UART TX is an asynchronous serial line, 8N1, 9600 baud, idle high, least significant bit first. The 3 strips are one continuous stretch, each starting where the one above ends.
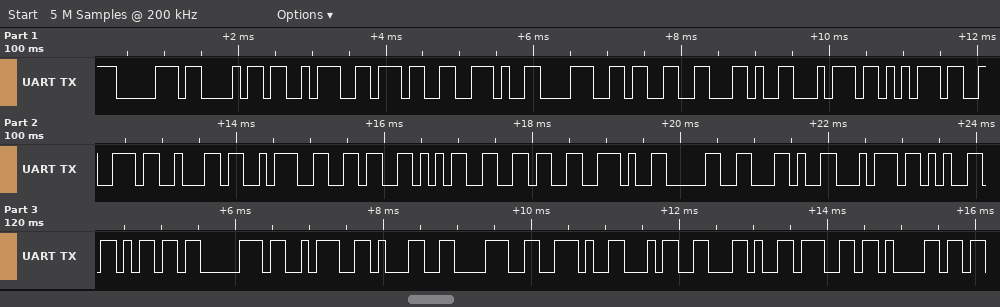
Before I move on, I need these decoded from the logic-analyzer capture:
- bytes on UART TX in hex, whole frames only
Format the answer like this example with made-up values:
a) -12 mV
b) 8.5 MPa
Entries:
a) 0x70 0x68 0x3A 0x37 0x2E 0x38 0x33 0x2C 0x74 0x75 0x72 0x62 0x3A 0x36 0x35 0x36 0x2E 0x30 0x2C 0x74 0x65 0x6D 0x70 0x3A 0x31 0x38 0x2E 0x34 0x2C 0x67 0x61
